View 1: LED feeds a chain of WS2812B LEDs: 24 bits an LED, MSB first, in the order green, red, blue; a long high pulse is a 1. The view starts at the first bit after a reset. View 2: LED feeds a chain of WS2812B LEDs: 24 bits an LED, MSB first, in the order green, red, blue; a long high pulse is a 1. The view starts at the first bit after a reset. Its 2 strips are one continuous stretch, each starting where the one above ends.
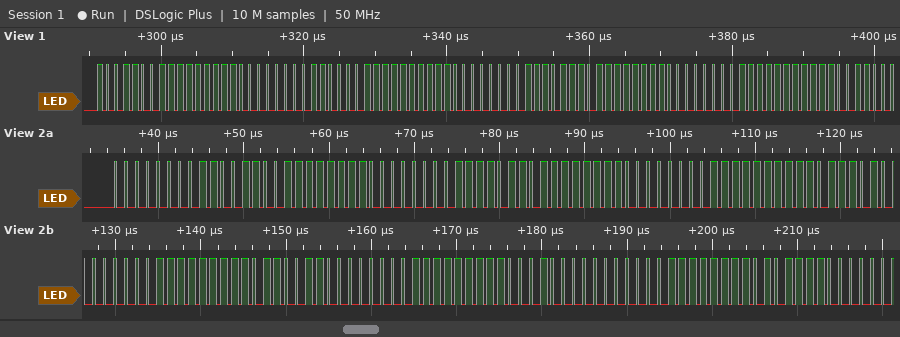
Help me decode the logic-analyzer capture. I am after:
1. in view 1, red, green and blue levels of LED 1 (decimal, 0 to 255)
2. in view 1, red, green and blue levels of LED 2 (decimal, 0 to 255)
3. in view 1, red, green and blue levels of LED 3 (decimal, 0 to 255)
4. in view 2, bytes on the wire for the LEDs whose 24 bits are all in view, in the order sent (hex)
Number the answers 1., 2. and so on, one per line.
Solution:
1. 255, 153, 0
2. 255, 195, 0
3. 255, 238, 0
4. 00 CC FF 00 F6 FF 00 FF DD 00 FF B3 00 FF 88 00 FF 5E
